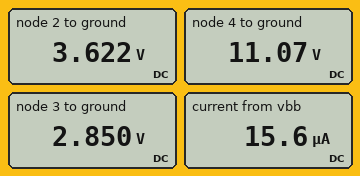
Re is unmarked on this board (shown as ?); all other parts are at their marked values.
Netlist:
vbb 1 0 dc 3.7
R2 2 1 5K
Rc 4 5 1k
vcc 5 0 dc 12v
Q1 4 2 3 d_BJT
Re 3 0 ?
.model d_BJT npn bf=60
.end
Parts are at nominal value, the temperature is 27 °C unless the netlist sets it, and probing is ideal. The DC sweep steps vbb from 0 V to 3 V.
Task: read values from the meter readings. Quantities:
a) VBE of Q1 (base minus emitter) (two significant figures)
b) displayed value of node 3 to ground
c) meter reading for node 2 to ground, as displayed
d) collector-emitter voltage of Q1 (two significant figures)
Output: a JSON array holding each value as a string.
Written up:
["770 mV", "2.850 V", "3.622 V", "8.2 V"]
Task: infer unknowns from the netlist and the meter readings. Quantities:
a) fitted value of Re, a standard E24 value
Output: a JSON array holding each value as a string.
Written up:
["3 kΩ"]
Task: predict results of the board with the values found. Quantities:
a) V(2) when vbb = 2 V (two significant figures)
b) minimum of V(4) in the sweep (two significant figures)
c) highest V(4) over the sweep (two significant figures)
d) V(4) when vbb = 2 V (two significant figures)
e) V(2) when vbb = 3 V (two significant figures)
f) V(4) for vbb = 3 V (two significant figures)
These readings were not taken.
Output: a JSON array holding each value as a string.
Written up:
["2.0 V", "11 V", "12 V", "12 V", "2.9 V", "11 V"]
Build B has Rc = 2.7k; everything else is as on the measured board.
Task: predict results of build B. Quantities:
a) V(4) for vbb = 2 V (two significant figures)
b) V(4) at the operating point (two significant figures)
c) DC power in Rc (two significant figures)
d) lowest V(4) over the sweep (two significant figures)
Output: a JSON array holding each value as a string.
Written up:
["11 V", "9.5 V", "2.4 mW", "10 V"]
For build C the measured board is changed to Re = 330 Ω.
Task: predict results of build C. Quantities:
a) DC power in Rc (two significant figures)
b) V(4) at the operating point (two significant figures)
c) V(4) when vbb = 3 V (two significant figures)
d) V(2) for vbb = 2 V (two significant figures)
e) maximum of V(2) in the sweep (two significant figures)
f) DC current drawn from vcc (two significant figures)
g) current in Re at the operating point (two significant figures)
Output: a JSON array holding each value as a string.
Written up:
["47 mW", "5.1 V", "6.8 V", "1.8 V", "2.6 V", "6.9 mA", "7.0 mA"]
